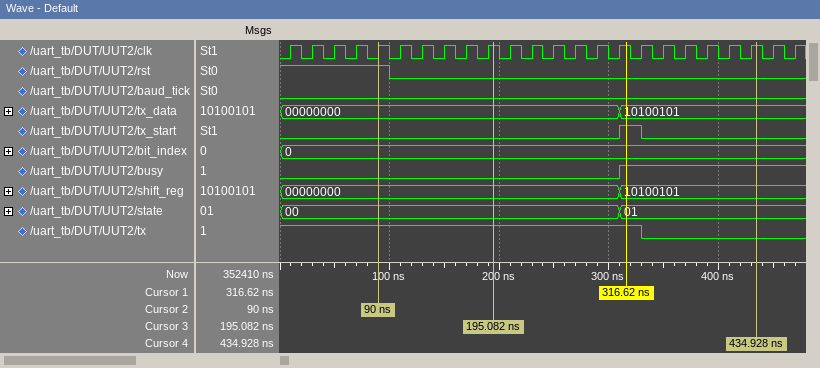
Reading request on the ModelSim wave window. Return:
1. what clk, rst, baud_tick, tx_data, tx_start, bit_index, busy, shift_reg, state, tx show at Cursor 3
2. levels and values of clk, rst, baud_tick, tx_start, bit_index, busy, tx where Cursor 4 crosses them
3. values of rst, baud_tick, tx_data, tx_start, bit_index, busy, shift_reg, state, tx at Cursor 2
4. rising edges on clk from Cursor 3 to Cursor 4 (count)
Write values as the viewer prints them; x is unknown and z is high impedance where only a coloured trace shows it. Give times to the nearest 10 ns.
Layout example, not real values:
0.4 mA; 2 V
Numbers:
clk=1, rst=0, baud_tick=0, tx_data=00000000, tx_start=0, bit_index=0, busy=0, shift_reg=00000000, state=00, tx=1; clk=1, rst=0, baud_tick=0, tx_start=0, bit_index=0, busy=1, tx=0; rst=1, baud_tick=0, tx_data=00000000, tx_start=0, bit_index=0, busy=0, shift_reg=00000000, state=00, tx=1; 12
